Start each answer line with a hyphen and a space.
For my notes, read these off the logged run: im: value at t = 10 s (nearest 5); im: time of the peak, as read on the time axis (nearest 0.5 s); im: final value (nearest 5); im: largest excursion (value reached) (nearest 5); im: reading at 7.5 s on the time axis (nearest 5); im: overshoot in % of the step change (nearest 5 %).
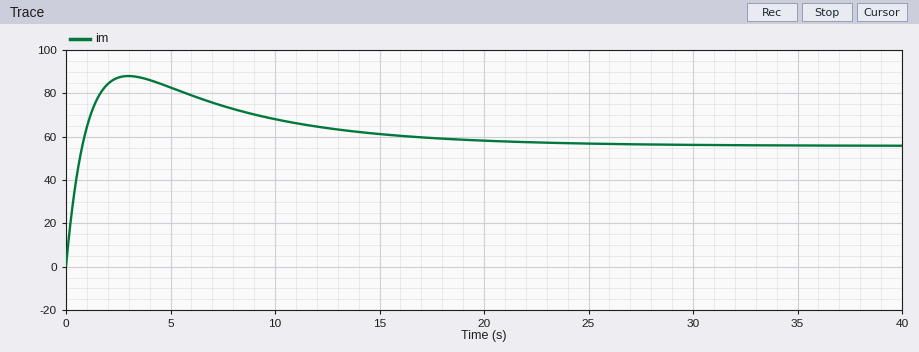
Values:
- 70
- 3.0 s
- 55
- 90
- 75
- 60 %
